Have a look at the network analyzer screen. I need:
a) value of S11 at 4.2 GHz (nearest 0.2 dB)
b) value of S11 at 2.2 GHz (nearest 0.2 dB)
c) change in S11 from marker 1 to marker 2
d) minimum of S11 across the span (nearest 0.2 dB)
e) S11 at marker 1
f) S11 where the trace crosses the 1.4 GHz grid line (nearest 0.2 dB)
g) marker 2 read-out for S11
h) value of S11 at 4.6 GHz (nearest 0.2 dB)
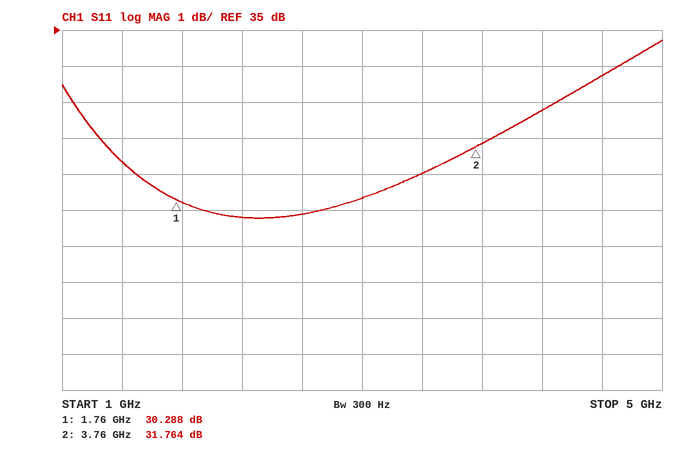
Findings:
32.8 dB
29.8 dB
1.476 dB
29.8 dB
30.288 dB
31.4 dB
31.764 dB
33.8 dB
